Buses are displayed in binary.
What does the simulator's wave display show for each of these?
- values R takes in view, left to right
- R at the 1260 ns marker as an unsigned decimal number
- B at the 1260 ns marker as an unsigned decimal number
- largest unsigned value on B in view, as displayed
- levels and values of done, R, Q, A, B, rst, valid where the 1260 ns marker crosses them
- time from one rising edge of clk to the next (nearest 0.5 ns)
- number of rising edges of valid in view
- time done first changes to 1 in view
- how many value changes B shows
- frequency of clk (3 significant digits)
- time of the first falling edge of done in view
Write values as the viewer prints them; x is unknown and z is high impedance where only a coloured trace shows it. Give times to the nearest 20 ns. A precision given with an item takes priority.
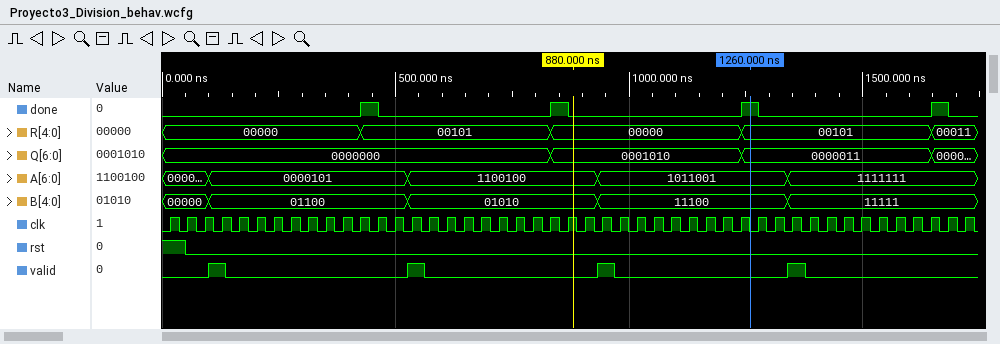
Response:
00000, 00101, 00000, 00101, 00011
5
28
11111
done=1, R=00101, Q=0000011, A=1011001, B=11100, rst=0, valid=0
37 ns
4
420 ns
4
27.0 MHz
460 ns
